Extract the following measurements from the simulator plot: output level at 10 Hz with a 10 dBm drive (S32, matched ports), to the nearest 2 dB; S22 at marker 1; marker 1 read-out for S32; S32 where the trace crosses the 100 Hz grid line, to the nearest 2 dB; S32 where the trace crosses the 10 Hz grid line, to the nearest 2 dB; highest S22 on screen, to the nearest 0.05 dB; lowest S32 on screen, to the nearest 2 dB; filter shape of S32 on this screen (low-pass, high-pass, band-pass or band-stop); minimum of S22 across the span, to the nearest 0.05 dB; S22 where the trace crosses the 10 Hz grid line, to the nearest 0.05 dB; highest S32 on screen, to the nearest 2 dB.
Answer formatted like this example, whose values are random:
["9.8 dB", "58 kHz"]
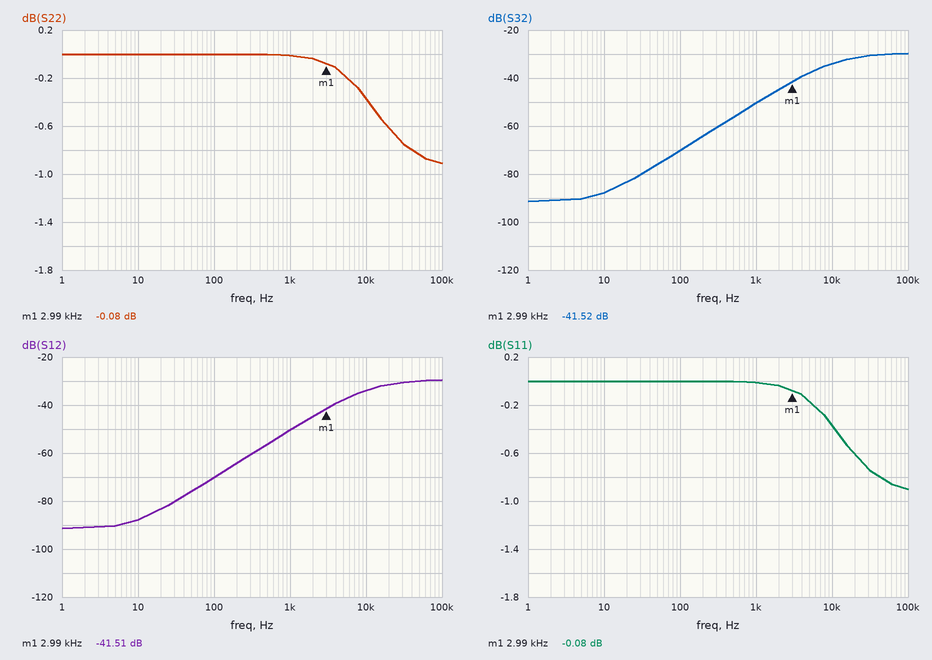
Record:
["-78 dBm", "-0.08 dB", "-41.52 dB", "-70 dB", "-88 dB", "0.00 dB", "-92 dB", "high-pass", "-0.90 dB", "0.00 dB", "-30 dB"]
